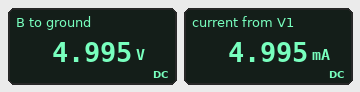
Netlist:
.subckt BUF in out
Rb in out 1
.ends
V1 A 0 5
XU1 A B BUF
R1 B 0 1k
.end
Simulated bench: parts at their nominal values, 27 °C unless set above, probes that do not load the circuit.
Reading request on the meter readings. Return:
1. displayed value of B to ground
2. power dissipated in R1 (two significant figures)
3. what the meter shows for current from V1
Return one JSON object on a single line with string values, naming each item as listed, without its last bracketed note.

{"displayed value of B to ground": "4.995 V", "power dissipated in R1": "25 mW", "what the meter shows for current from V1": "4.995 mA"}
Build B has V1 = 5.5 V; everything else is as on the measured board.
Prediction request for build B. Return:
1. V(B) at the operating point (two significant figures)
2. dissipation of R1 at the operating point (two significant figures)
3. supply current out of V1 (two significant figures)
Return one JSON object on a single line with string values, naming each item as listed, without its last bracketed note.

{"V(B) at the operating point": "5.5 V", "dissipation of R1 at the operating point": "30 mW", "supply current out of V1": "5.5 mA"}
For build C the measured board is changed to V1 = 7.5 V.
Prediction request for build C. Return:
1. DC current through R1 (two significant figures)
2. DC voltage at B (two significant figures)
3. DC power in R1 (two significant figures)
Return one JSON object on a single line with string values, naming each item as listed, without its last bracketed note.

{"DC current through R1": "7.5 mA", "DC voltage at B": "7.5 V", "DC power in R1": "56 mW"}
